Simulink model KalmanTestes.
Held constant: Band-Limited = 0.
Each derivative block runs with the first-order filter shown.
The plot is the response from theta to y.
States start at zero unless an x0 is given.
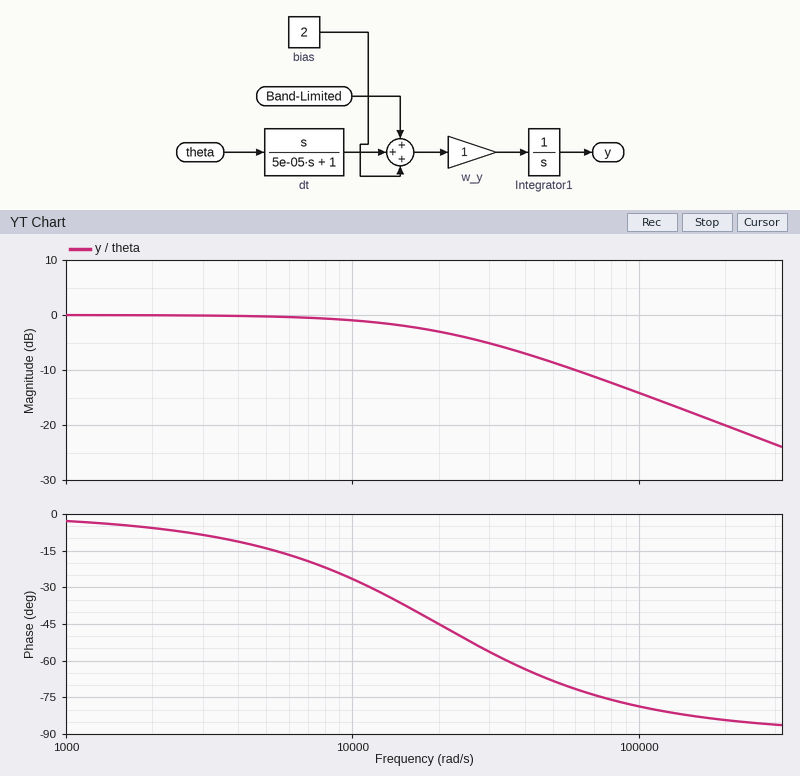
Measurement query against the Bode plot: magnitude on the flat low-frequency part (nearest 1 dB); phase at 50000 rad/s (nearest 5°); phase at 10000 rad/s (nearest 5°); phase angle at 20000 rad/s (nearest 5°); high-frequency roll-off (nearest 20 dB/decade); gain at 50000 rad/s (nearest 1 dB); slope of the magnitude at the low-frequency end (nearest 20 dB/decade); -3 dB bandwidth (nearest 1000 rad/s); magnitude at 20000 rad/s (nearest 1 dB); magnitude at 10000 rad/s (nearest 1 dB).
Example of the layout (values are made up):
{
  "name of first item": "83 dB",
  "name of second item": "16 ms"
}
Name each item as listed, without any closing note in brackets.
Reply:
{
  "magnitude on the flat low-frequency part": "0 dB",
  "phase at 50000 rad/s": "-70°",
  "phase at 10000 rad/s": "-25°",
  "phase angle at 20000 rad/s": "-45°",
  "high-frequency roll-off": "-20 dB/decade",
  "gain at 50000 rad/s": "-9 dB",
  "slope of the magnitude at the low-frequency end": "0 dB/decade",
  "-3 dB bandwidth": "20000 rad/s",
  "magnitude at 20000 rad/s": "-3 dB",
  "magnitude at 10000 rad/s": "-1 dB"
}
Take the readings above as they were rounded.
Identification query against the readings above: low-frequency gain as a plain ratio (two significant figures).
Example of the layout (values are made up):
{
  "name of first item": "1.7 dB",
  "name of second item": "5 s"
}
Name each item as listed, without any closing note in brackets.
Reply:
{
  "low-frequency gain as a plain ratio": "1.0"
}
